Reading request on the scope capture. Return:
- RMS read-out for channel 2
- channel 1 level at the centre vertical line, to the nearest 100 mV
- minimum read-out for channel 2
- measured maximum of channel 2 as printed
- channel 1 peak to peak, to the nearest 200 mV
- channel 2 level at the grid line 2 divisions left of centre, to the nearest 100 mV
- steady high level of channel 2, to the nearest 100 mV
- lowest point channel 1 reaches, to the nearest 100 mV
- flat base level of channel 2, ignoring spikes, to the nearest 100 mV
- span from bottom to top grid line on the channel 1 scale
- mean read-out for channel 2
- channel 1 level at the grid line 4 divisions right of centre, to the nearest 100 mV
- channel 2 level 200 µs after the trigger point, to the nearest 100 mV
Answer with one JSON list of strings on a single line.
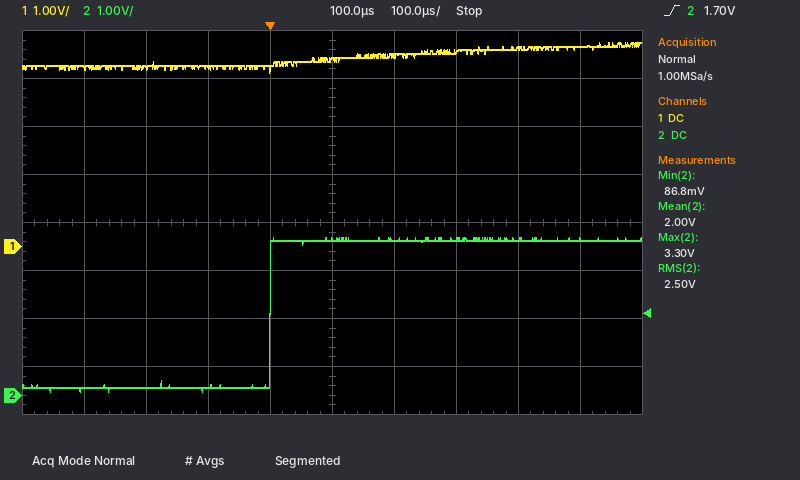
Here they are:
["2.50 V", "3.9 V", "86.8 mV", "3.30 V", "600 mV", "200 mV", "3.2 V", "3.6 V", "200 mV", "8 V", "2.00 V", "4.2 V", "3.2 V"]
